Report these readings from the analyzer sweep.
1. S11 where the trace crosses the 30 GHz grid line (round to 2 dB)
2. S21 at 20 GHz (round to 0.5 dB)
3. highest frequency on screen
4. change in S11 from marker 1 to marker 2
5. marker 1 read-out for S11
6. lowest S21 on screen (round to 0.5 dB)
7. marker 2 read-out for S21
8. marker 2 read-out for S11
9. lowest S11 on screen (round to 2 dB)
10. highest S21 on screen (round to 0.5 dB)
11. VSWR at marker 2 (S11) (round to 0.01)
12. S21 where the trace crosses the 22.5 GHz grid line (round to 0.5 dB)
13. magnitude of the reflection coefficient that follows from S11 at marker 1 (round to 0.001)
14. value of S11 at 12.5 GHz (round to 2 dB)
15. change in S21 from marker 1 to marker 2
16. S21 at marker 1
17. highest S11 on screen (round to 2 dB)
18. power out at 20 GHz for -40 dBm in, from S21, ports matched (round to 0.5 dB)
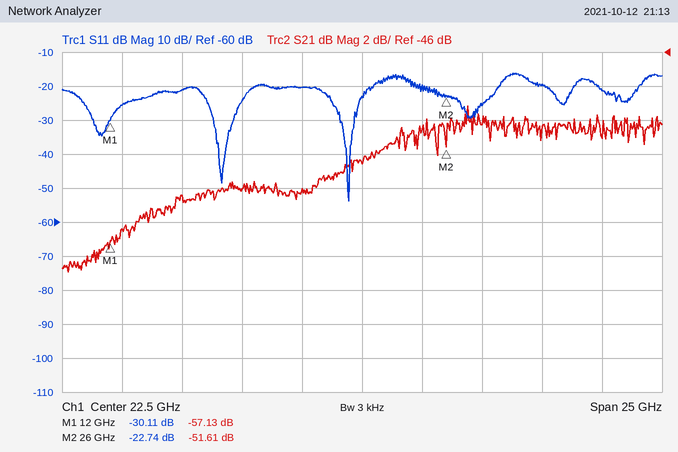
-20 dB
-54.0 dB
35 GHz
7.37 dB
-30.11 dB
-59.0 dB
-51.61 dB
-22.74 dB
-54 dB
-49.0 dB
1.16
-52.5 dB
0.031
-26 dB
5.52 dB
-57.13 dB
-16 dB
-94.0 dBm
